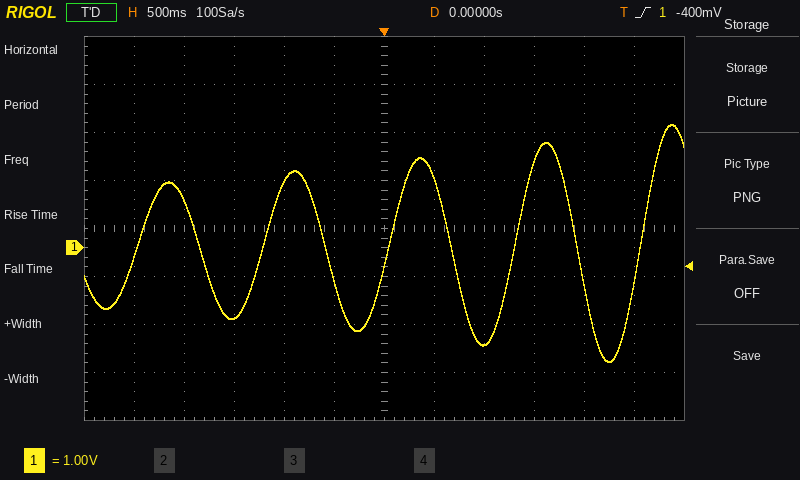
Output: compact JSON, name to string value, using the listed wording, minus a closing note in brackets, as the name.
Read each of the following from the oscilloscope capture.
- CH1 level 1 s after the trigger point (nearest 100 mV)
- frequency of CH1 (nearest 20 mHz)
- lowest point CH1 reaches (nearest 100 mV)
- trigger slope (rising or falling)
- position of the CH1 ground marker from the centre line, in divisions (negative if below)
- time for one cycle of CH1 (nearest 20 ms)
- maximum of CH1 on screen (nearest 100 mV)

{"CH1 level 1 s after the trigger point": "-2.0 V", "frequency of CH1": "800 mHz", "lowest point CH1 reaches": "-2.4 V", "trigger slope": "rising", "position of the CH1 ground marker from the centre line, in divisions": "-0.4 div", "time for one cycle of CH1": "1.26 s", "maximum of CH1 on screen": "2.6 V"}
